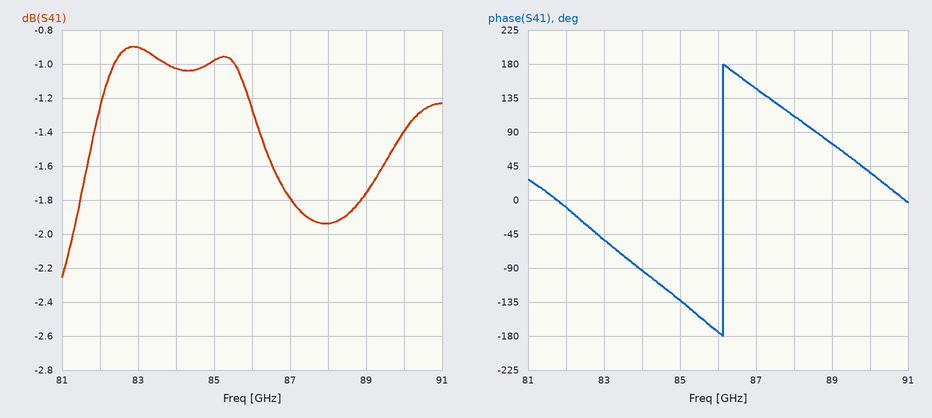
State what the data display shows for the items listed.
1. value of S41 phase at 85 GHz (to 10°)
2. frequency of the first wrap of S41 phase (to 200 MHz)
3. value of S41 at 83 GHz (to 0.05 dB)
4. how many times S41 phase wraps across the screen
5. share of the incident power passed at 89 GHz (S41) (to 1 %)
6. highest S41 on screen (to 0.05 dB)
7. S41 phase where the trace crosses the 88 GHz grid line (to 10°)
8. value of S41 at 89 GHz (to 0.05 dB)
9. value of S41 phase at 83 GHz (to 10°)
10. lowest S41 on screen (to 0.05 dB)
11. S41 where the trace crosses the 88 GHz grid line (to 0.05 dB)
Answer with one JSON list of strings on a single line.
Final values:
["-130°", "86.2 GHz", "-0.90 dB", "1", "67 %", "-0.90 dB", "110°", "-1.75 dB", "-50°", "-2.25 dB", "-1.95 dB"]
